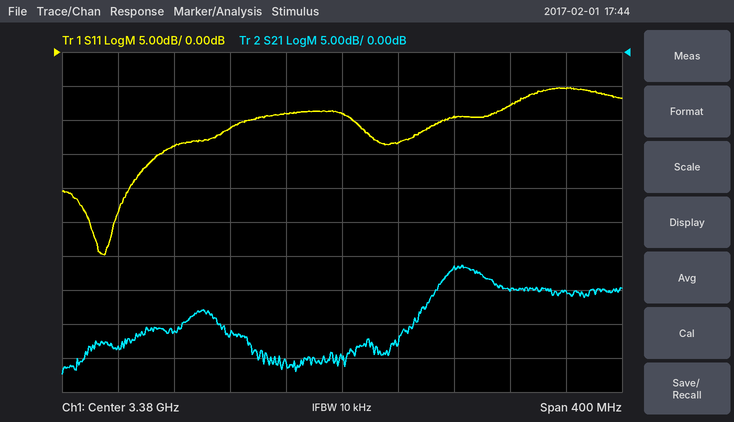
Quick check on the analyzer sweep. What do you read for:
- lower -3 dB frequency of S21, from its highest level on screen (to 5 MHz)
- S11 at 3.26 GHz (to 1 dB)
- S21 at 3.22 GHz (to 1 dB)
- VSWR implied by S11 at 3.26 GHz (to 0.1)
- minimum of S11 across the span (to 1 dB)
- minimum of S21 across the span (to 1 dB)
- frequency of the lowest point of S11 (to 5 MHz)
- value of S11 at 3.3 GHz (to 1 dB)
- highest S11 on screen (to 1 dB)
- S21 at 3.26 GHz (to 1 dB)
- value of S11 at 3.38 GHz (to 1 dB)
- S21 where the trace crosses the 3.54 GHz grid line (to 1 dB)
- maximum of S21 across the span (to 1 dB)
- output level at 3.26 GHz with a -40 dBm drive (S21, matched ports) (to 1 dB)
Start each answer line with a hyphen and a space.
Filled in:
- 3.450 GHz
- -14 dB
- -43 dB
- 1.5
- -30 dB
- -47 dB
- 3.210 GHz
- -11 dB
- -5 dB
- -41 dB
- -9 dB
- -35 dB
- -31 dB
- -81 dBm
